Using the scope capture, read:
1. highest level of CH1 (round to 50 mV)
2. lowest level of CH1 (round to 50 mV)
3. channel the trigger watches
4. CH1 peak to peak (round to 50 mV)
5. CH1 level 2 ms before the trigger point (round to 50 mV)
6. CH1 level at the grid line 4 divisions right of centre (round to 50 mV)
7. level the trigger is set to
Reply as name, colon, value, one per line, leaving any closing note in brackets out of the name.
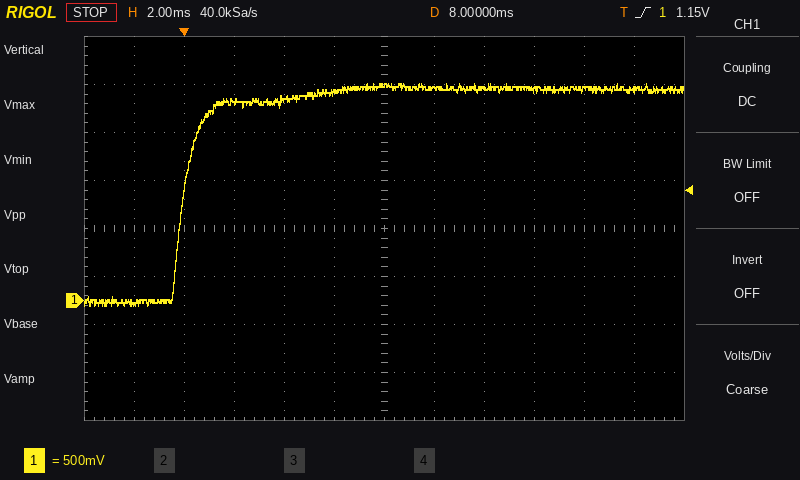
highest level of CH1: 2.25 V
lowest level of CH1: -50 mV
channel the trigger watches: CH1
CH1 peak to peak: 2.30 V
CH1 level 2 ms before the trigger point: 0 mV
CH1 level at the grid line 4 divisions right of centre: 2.20 V
level the trigger is set to: 1.15 V
